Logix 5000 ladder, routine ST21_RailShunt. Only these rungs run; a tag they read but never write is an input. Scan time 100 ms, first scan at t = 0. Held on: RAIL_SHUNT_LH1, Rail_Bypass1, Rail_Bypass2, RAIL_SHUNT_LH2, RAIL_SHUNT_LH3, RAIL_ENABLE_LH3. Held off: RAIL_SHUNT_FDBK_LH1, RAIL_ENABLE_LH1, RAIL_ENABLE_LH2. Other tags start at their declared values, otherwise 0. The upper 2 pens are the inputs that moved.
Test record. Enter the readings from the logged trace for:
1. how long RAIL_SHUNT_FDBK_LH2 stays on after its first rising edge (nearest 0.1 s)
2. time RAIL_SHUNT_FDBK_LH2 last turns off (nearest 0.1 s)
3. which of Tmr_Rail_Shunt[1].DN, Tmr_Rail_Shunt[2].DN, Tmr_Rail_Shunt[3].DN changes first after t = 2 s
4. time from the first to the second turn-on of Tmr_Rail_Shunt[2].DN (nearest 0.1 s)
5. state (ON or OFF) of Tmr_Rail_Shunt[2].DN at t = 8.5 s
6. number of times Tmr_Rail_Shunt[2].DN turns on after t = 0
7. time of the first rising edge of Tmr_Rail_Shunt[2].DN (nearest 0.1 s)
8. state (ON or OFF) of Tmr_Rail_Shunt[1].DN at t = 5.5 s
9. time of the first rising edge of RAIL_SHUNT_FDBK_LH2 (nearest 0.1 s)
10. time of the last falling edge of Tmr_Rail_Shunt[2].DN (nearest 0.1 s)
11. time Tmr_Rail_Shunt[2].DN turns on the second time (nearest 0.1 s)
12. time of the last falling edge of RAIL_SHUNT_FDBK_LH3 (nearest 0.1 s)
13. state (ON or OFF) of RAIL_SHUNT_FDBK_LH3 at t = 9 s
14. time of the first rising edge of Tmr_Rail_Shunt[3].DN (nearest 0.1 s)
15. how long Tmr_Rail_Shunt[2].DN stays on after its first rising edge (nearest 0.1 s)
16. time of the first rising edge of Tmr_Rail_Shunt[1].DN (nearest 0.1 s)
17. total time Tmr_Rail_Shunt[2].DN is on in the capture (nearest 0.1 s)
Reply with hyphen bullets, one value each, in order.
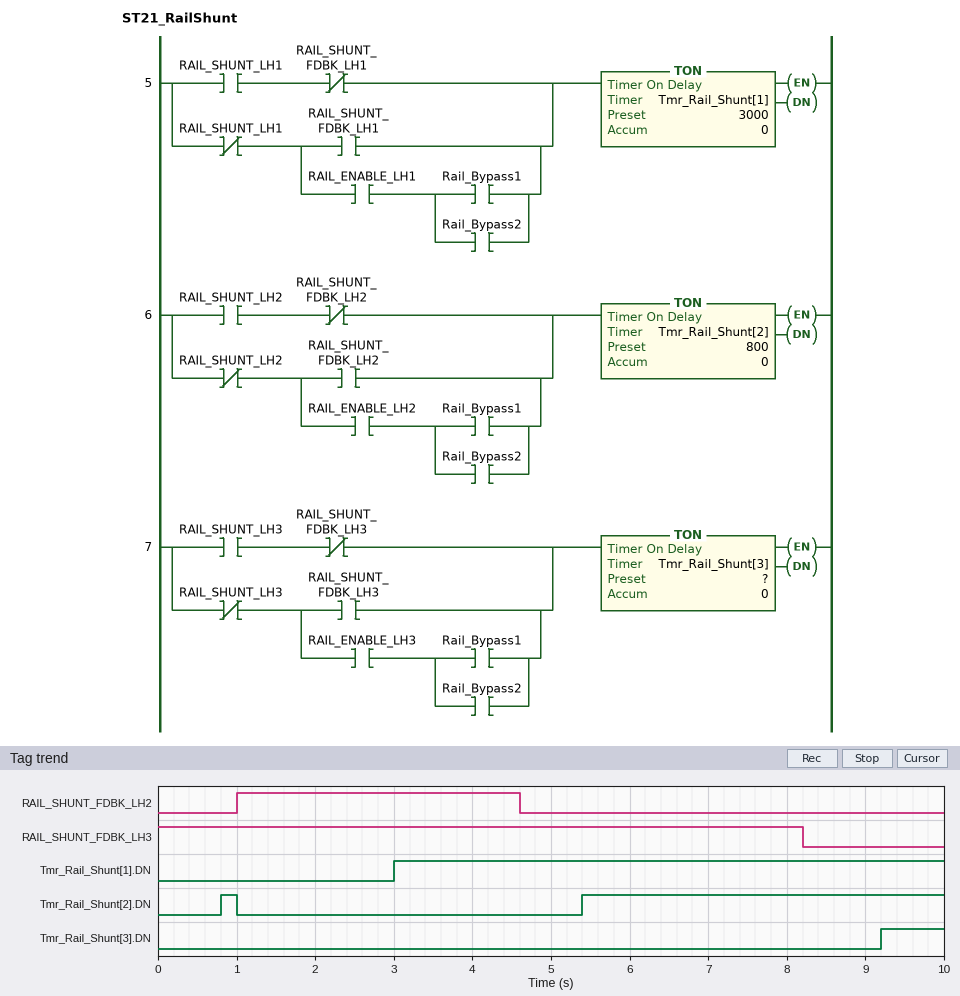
- 3.6 s
- 4.6 s
- Tmr_Rail_Shunt[1].DN
- 4.6 s
- ON
- 2
- 0.8 s
- ON
- 1.0 s
- 1.0 s
- 5.4 s
- 8.2 s
- OFF
- 9.2 s
- 0.2 s
- 3.0 s
- 4.8 s
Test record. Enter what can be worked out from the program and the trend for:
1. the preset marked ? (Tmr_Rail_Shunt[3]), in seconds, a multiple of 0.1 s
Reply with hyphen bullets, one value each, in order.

- 1.0 s
